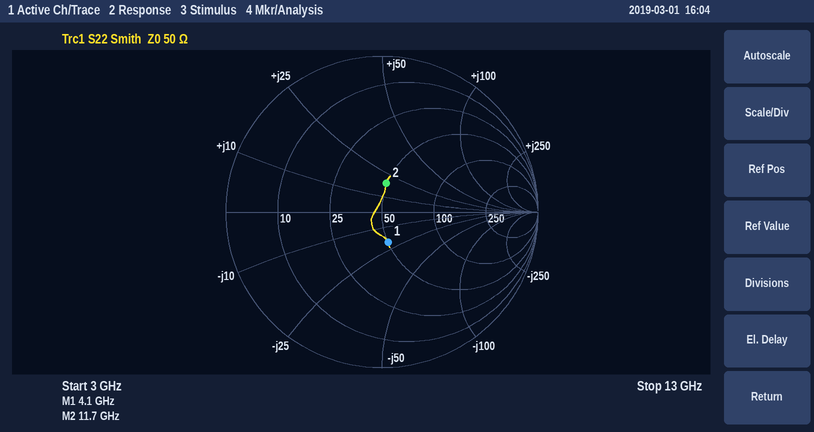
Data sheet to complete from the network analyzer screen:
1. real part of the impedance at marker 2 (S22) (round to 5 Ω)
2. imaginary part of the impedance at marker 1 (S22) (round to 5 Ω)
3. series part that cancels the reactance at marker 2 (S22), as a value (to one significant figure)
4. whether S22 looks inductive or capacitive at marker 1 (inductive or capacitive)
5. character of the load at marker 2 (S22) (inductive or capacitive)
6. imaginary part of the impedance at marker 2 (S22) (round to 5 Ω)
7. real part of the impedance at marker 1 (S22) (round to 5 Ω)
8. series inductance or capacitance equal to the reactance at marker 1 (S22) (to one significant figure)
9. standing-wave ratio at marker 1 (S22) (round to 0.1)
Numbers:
50 Ω
-20 Ω
700 fF
capacitive
inductive
+20 Ω
50 Ω
2 pF
1.5
